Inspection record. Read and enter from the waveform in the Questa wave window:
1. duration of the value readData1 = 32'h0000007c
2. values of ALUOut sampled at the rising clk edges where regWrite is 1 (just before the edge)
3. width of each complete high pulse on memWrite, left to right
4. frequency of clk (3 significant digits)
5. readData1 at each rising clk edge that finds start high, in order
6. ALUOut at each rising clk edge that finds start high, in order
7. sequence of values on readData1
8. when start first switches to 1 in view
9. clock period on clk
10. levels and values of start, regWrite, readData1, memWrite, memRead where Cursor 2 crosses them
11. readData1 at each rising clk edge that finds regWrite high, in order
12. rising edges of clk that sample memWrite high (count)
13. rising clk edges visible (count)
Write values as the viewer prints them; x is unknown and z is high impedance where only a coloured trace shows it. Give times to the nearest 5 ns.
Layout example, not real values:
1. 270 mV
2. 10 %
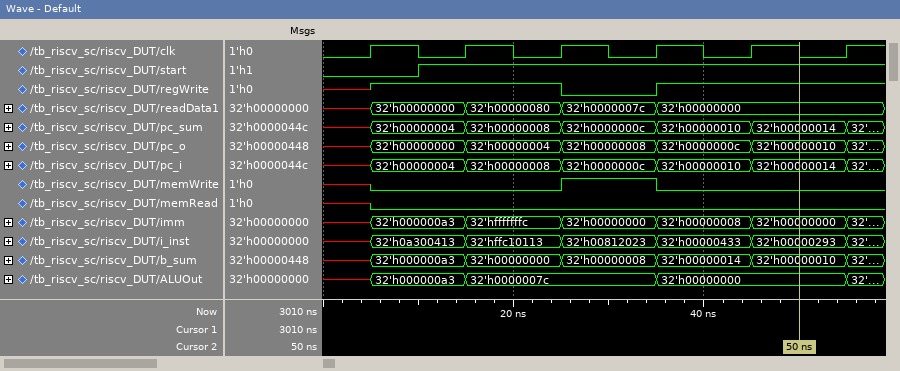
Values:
1. 10 ns
2. 32'h000000a3, 32'h0000007c, 32'h00000000, 32'h00000000
3. 10 ns
4. 100 MHz
5. 32'h00000000, 32'h00000080, 32'h0000007c, 32'h00000000, 32'h00000000
6. 32'h000000a3, 32'h0000007c, 32'h0000007c, 32'h00000000, 32'h00000000
7. x, 32'h00000000, 32'h00000080, 32'h0000007c, 32'h00000000
8. 10 ns
9. 10 ns
10. start=1, regWrite=1, readData1=32'h00000000, memWrite=0, memRead=0
11. 32'h00000000, 32'h00000080, 32'h00000000, 32'h00000000
12. 1
13. 6
